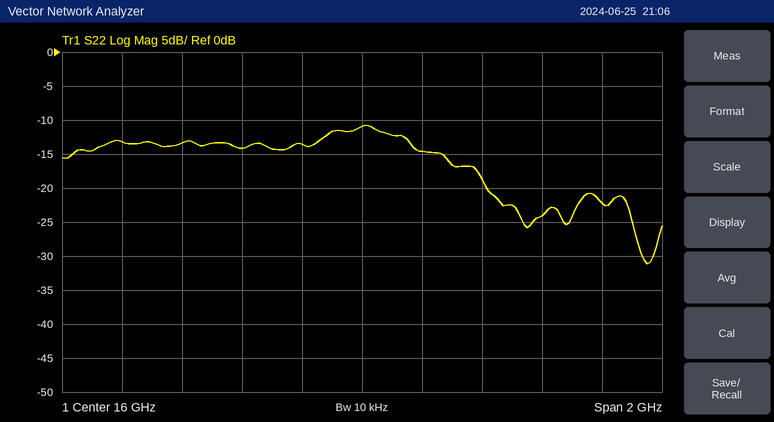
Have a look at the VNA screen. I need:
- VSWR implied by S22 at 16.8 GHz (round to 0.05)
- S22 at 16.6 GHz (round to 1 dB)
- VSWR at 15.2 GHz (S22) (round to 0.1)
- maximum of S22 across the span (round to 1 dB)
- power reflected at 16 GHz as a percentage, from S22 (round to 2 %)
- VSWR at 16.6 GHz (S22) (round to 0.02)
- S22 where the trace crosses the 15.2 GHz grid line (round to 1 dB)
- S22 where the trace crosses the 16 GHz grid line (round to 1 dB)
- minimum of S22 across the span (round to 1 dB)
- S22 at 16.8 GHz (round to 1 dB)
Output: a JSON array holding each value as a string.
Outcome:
["1.15", "-24 dB", "1.6", "-11 dB", "8 %", "1.14", "-13 dB", "-11 dB", "-31 dB", "-22 dB"]
